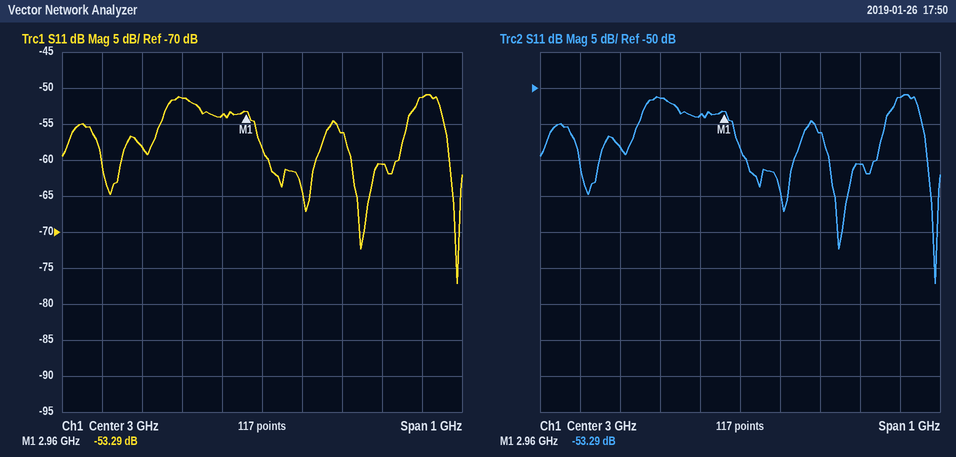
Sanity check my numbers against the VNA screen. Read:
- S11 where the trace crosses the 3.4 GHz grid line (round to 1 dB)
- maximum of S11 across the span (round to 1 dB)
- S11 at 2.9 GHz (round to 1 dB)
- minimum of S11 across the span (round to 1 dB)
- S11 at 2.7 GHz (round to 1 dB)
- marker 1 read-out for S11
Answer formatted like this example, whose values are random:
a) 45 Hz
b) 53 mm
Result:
a) -51 dB
b) -51 dB
c) -54 dB
d) -77 dB
e) -58 dB
f) -53.29 dB
